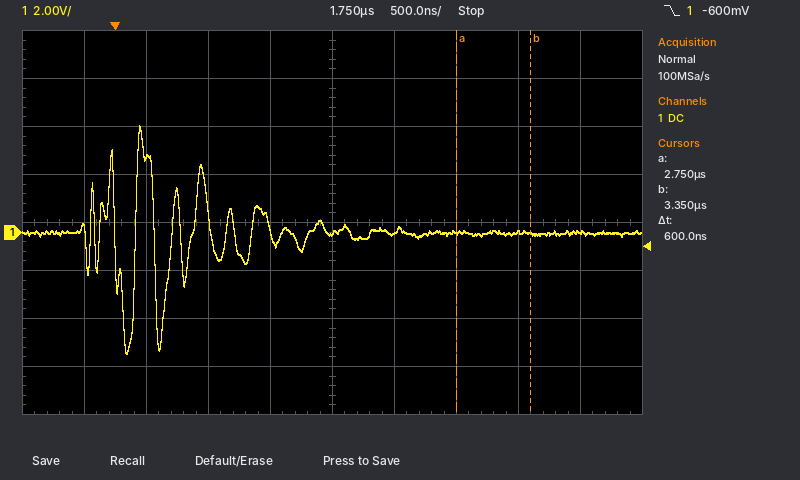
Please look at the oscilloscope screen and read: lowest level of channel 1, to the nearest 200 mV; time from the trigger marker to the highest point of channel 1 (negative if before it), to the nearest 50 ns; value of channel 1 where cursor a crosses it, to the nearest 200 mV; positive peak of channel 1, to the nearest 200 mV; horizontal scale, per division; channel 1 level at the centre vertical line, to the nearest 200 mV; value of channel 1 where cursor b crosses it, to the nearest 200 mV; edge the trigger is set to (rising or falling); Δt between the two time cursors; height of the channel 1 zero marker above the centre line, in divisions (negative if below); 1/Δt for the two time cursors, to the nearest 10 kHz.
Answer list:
-5.0 V
+200 ns
0.0 V
4.4 V
500 ns
0.0 V
0.0 V
falling
600 ns
-0.2 div
1.67 MHz
